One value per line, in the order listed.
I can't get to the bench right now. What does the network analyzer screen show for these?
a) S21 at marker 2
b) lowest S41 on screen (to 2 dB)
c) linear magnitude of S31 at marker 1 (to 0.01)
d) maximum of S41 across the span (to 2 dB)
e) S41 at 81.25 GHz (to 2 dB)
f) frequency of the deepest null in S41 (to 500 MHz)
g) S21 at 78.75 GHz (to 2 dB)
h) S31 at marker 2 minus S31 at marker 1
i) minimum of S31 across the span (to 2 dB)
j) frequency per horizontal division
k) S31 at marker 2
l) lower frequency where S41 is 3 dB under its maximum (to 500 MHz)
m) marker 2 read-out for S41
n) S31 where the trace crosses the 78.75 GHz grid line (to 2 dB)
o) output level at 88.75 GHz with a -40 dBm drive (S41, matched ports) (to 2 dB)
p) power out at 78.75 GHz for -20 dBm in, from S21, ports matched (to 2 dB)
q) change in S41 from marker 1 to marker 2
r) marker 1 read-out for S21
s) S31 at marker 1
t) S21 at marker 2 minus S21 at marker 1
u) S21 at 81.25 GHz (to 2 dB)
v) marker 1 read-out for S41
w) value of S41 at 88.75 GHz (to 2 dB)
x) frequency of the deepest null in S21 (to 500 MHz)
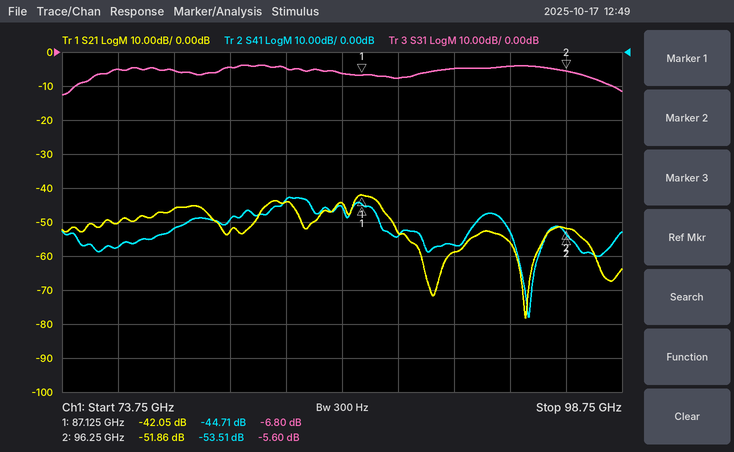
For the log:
-51.86 dB
-78 dB
0.46
-42 dB
-50 dB
94.5 GHz
-46 dB
1.20 dB
-12 dB
2.5 GHz
-5.60 dB
83.0 GHz
-53.51 dB
-6 dB
-94 dBm
-66 dBm
-8.80 dB
-42.05 dB
-6.80 dB
-9.81 dB
-52 dB
-44.71 dB
-54 dB
94.5 GHz
